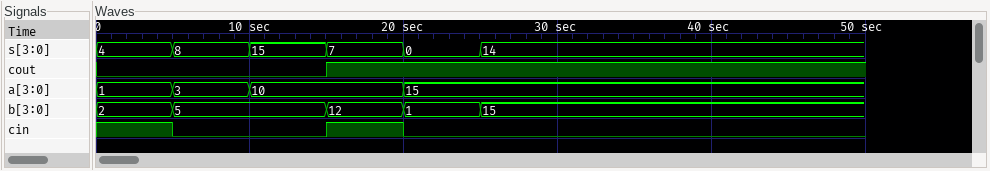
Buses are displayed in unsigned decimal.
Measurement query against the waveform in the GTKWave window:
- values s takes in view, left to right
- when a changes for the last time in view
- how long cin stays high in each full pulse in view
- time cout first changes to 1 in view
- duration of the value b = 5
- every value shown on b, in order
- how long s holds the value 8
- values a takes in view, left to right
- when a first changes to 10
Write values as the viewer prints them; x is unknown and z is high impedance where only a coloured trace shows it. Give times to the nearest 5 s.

4, 8, 15, 7, 0, 14
20 s
5 s
15 s
10 s
2, 5, 12, 1, 15
5 s
1, 3, 10, 15
10 s
